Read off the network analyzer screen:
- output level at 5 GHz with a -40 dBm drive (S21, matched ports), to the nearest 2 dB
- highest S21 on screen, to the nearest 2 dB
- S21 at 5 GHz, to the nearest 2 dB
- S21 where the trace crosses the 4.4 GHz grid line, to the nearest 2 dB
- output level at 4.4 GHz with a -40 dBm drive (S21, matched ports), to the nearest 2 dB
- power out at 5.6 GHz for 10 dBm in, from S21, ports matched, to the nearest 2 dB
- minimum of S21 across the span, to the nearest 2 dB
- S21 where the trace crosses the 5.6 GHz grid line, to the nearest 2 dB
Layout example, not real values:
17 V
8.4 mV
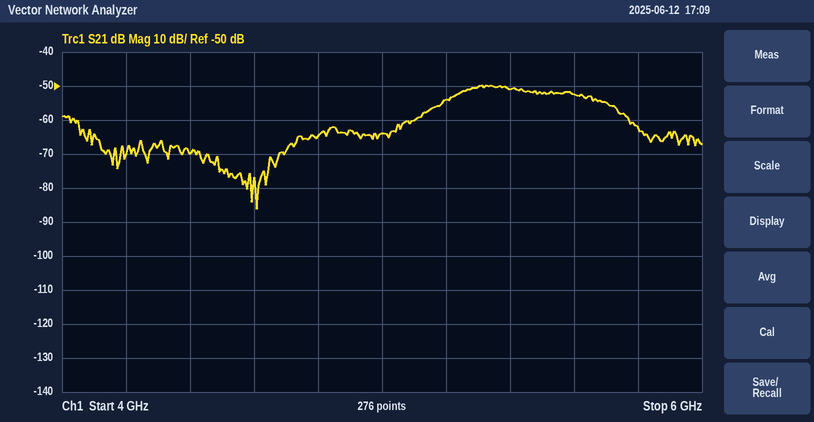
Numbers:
-104 dBm
-50 dB
-64 dB
-70 dB
-110 dBm
-42 dBm
-86 dB
-52 dB
